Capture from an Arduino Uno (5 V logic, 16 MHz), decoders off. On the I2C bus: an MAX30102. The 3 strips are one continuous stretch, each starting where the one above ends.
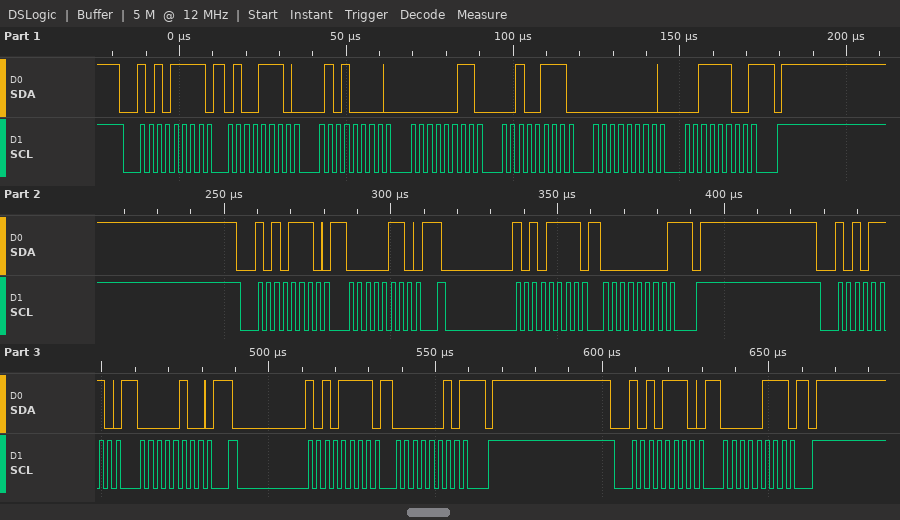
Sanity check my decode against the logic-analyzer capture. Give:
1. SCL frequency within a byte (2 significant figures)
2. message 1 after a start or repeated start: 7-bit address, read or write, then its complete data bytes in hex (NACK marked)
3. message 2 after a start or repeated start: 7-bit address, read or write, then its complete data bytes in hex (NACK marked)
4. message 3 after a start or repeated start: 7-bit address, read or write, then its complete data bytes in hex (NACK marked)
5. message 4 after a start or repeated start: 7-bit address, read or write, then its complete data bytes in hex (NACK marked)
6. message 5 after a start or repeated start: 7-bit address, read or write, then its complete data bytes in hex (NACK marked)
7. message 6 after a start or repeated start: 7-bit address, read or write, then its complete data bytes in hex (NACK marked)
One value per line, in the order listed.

400 kHz
0x57 read: 4E 50 03 27 00 3C NACK
0x57 write: 06
0x57 read: 00 NACK
0x57 write: 04
0x57 read: 02 NACK
0x57 write: 07
